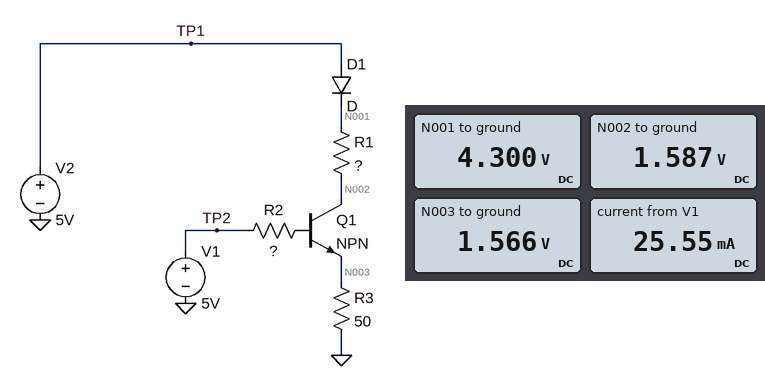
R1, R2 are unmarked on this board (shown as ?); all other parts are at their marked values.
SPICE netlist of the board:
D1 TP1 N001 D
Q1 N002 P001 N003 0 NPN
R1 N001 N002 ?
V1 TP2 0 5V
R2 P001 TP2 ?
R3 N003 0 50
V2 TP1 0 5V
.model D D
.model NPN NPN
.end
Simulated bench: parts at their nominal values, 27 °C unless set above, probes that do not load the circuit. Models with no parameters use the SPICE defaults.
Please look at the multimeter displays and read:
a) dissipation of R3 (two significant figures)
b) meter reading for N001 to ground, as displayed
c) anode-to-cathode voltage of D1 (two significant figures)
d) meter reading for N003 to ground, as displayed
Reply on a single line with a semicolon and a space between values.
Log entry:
49 mW; 4.300 V; 700 mV; 1.566 V
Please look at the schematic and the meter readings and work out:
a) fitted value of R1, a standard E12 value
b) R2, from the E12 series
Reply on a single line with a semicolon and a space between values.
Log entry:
470 Ω; 100 Ω
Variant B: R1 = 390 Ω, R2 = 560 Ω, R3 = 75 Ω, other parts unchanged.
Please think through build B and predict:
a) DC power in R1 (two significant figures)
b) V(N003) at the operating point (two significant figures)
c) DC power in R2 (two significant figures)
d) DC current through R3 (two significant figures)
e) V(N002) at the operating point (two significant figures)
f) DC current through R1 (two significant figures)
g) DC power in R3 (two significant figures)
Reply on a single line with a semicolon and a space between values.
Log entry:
27 mW; 1.0 V; 17 mW; 14 mA; 1.1 V; 8.3 mA; 14 mW
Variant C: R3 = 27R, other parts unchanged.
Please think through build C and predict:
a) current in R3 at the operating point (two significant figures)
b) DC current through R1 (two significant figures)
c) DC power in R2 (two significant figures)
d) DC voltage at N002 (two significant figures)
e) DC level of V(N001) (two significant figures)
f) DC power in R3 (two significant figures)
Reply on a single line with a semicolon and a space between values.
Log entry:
38 mA; 6.9 mA; 96 mW; 1.0 V; 4.3 V; 39 mW
